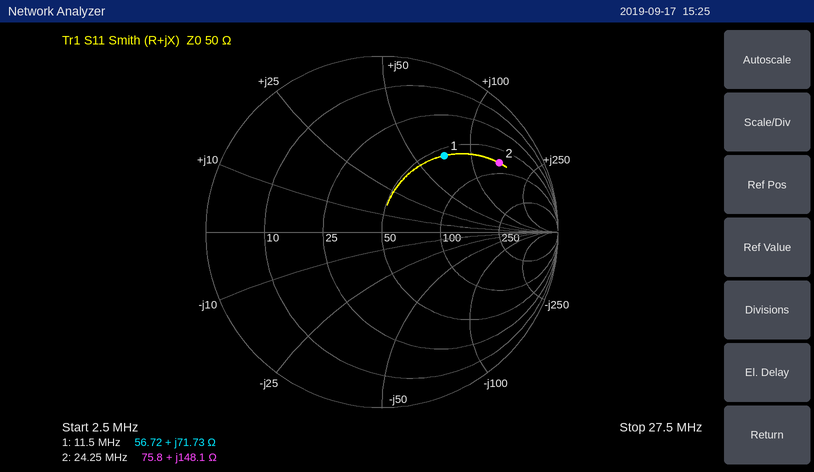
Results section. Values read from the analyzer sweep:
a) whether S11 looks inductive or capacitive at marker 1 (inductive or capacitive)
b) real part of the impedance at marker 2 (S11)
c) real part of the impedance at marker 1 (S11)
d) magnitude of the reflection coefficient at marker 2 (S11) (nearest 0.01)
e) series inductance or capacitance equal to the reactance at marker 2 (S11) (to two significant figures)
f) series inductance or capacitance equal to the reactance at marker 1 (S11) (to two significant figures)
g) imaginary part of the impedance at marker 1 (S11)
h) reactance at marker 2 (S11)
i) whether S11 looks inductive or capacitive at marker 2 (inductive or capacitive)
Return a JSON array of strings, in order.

["inductive", "75.8 Ω", "56.72 Ω", "0.77", "970 nH", "990 nH", "+71.73 Ω", "+148.1 Ω", "inductive"]
